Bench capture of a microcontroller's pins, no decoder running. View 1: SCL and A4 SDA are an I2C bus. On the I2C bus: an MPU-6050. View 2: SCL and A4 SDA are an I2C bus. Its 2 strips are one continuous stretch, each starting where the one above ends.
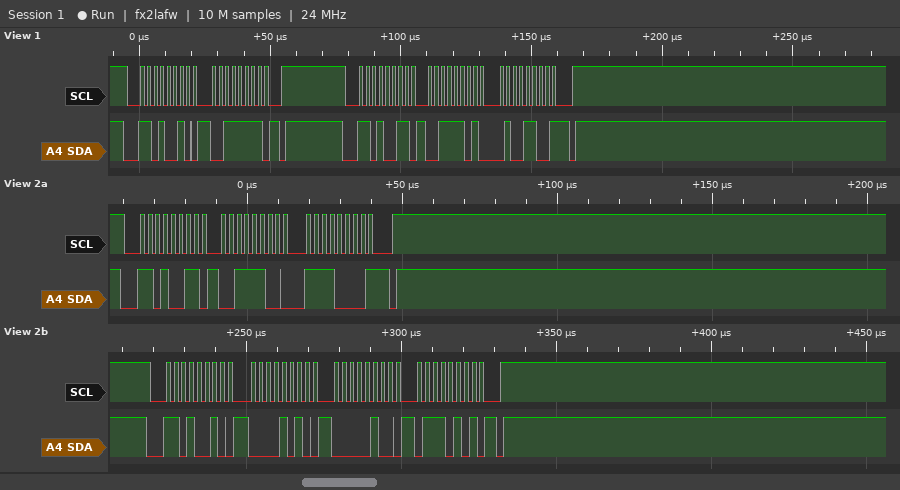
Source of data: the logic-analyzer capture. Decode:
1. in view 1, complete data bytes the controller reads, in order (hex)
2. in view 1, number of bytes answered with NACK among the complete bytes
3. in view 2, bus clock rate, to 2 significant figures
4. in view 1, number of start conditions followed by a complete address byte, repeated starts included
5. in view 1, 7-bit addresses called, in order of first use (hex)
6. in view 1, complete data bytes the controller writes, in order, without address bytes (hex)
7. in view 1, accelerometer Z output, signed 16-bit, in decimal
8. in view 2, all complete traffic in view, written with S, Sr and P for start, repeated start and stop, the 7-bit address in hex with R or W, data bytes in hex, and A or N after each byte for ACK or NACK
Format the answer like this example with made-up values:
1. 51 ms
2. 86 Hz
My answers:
1. 3D 4C
2. 1
3. 400 kHz
4. 2
5. 0x69
6. 3F
7. 15692
8. S 69R A 3C A F0 N P S 69W A 0A A 04 A 75 A P
